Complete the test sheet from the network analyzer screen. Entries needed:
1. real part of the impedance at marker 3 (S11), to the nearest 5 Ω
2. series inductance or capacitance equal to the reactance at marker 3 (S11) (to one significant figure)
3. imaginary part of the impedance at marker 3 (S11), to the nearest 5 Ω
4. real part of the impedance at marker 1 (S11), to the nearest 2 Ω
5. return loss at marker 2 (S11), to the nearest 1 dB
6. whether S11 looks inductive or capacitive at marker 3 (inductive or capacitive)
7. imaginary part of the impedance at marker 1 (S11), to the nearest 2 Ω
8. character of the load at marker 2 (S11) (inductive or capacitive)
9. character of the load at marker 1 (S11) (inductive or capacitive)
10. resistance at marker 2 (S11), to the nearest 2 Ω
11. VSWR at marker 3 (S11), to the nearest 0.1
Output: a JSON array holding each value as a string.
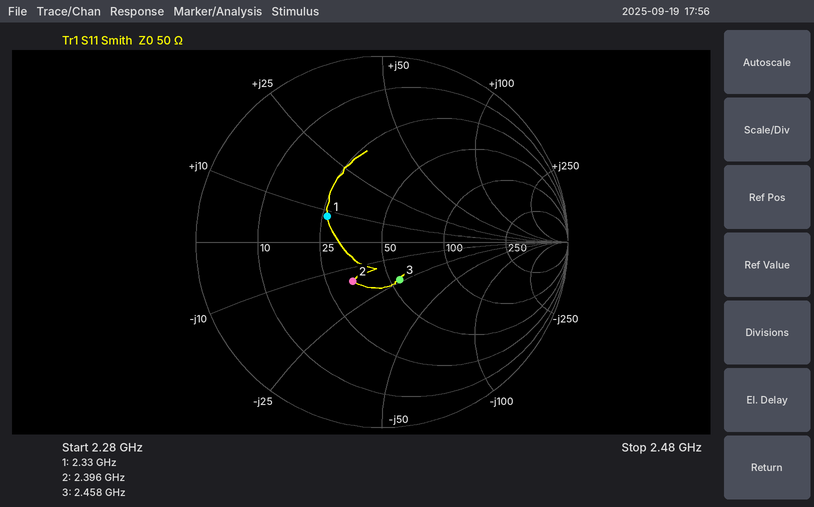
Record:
["55 Ω", "3 pF", "-25 Ω", "26 Ω", "12 dB", "capacitive", "+8 Ω", "capacitive", "inductive", "34 Ω", "1.6"]
